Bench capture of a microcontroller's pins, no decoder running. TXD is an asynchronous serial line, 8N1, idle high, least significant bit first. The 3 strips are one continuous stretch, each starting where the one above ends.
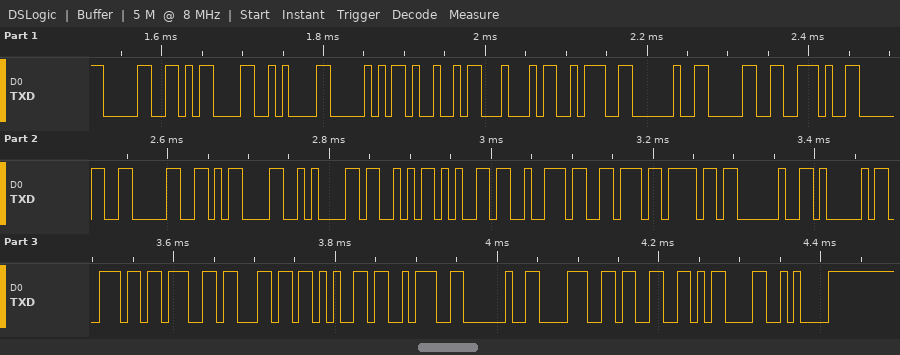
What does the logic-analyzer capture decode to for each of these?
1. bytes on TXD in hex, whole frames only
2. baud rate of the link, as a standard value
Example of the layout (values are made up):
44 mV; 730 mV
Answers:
30 0D 0A 50 49 44 3A 20 30 2E 30 30 0D 0A 53 65 72 76 6F 20 41 6E 67 6C 65 3A 20 38 33 0D 0A; 115200 baud
